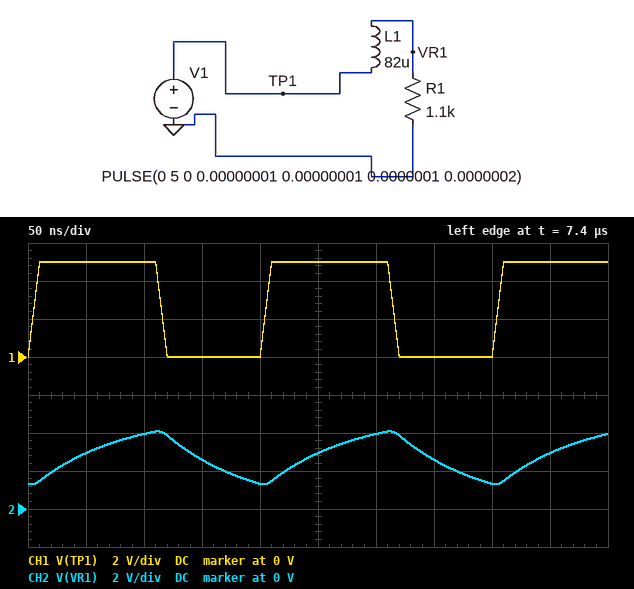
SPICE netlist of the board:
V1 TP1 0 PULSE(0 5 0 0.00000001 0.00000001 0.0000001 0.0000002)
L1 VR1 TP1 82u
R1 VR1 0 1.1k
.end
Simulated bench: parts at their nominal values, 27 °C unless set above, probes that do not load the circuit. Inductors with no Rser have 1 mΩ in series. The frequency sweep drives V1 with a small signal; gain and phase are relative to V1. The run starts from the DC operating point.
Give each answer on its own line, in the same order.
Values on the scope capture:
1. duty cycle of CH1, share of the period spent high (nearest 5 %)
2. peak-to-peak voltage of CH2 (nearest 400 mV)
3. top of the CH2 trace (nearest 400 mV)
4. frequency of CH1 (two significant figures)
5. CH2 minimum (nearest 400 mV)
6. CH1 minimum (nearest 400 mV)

55 %
2.8 V
4.0 V
5.0 MHz
1.2 V
0 V
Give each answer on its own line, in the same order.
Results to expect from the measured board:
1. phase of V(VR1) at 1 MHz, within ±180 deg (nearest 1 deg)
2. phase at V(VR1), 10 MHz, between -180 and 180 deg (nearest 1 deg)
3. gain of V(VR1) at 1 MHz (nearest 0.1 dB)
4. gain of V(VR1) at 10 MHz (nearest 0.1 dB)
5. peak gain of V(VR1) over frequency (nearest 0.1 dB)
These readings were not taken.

-25 deg
-78 deg
-0.9 dB
-13.6 dB
0 dB
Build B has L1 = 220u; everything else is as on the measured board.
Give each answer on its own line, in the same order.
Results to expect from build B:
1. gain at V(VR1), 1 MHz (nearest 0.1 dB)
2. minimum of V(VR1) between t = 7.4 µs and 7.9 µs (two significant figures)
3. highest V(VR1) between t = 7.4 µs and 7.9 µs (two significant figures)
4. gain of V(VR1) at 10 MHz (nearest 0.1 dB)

-4.1 dB
2.2 V
3.3 V
-22.0 dB
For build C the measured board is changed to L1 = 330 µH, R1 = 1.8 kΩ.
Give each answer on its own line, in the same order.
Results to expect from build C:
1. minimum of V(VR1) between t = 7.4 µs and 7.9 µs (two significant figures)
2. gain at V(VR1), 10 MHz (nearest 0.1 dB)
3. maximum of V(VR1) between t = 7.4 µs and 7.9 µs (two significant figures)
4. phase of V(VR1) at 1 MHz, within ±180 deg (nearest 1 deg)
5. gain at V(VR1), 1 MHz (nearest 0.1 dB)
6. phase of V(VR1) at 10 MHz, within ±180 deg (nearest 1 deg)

2.1 V
-21.3 dB
3.4 V
-49 deg
-3.7 dB
-85 deg
